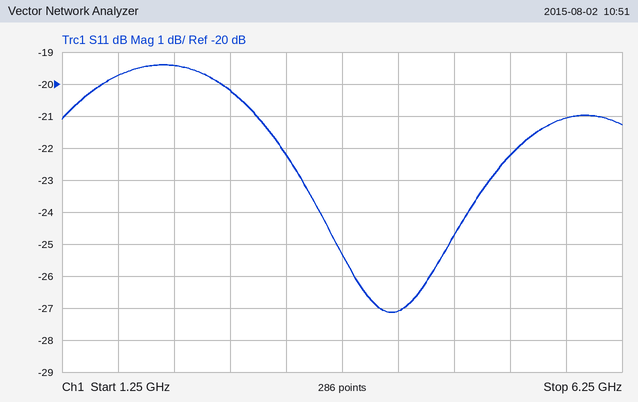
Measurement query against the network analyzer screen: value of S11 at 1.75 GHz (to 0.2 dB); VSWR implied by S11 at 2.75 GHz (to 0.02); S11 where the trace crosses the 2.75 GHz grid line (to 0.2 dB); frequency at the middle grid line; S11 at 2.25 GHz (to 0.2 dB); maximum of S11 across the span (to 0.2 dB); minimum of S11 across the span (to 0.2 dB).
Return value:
-19.8 dB
1.22
-20.2 dB
3.75 GHz
-19.4 dB
-19.4 dB
-27.2 dB
